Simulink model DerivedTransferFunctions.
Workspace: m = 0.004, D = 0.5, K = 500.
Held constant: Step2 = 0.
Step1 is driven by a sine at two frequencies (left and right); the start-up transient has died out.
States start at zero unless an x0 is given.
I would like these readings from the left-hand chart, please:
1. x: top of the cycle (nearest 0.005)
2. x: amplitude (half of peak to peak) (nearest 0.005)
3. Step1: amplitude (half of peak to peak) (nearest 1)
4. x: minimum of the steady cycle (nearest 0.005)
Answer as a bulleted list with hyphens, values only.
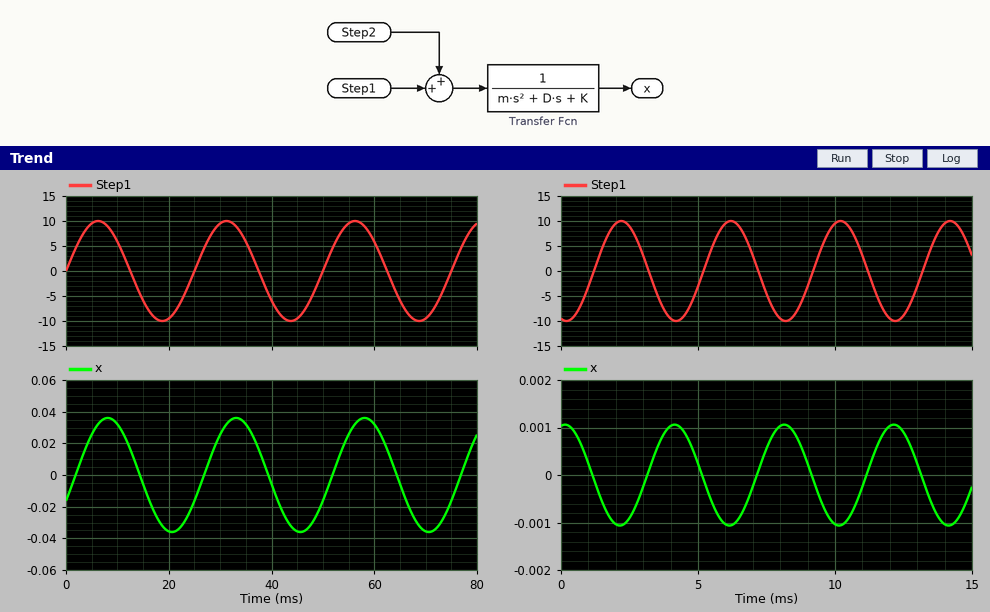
- 0.035
- 0.035
- 10
- -0.035
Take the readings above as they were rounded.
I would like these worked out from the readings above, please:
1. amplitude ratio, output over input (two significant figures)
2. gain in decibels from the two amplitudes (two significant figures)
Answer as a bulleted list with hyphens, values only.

- 0.0035
- -49 dB
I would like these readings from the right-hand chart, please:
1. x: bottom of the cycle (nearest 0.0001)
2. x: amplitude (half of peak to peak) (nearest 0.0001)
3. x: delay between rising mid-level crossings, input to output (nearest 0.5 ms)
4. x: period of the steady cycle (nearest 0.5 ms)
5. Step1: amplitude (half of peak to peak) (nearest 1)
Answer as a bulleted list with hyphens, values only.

- -0.0011
- 0.0011
- 2.0 ms
- 4.0 ms
- 10
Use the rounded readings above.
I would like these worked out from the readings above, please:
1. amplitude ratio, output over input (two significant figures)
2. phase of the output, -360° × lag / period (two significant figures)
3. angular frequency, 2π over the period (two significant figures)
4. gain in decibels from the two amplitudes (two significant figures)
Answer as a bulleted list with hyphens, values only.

- 0.00011
- -180°
- 1.6 rad/ms
- -79 dB
